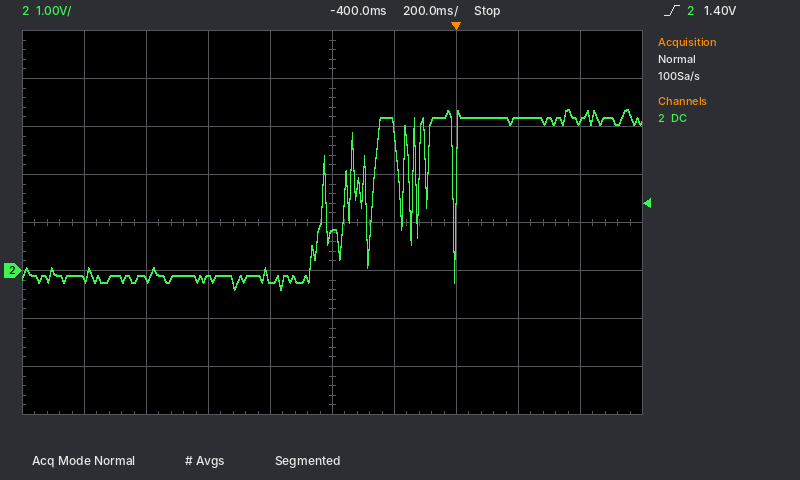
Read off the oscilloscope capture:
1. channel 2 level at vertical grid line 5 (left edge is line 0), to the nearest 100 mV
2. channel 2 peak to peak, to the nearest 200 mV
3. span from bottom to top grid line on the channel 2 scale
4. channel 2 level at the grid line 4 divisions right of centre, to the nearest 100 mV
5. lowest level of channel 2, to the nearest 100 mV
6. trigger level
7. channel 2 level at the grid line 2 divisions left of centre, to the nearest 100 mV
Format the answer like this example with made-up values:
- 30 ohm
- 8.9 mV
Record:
- 800 mV
- 3.8 V
- 8 V
- 3.1 V
- -400 mV
- 1.40 V
- -100 mV
